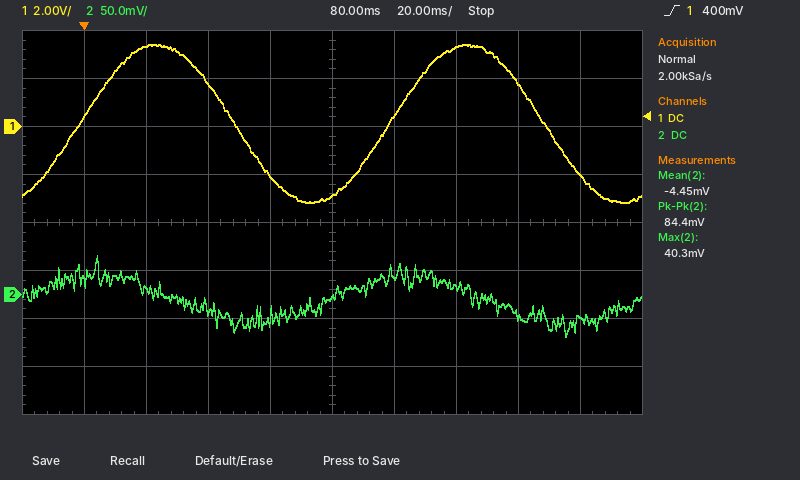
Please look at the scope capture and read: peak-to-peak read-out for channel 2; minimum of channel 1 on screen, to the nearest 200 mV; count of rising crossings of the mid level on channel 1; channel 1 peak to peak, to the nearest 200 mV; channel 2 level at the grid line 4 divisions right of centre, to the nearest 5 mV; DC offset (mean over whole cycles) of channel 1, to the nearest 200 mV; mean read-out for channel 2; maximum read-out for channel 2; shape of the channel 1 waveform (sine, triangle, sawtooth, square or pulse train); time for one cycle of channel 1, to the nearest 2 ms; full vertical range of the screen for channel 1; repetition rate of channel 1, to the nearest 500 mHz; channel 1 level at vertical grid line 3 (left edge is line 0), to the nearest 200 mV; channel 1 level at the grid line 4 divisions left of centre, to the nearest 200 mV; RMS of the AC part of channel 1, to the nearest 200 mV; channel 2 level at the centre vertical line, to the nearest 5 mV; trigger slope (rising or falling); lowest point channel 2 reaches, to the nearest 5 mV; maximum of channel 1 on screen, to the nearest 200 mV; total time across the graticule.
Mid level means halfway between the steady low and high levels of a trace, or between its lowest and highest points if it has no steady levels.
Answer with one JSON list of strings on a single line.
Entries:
["84.4 mV", "-3.2 V", "2", "6.6 V", "-25 mV", "200 mV", "-4.45 mV", "40.3 mV", "sine", "100 ms", "16 V", "10.0 Hz", "1.8 V", "400 mV", "2.4 V", "-5 mV", "rising", "-45 mV", "3.4 V", "200 ms"]
